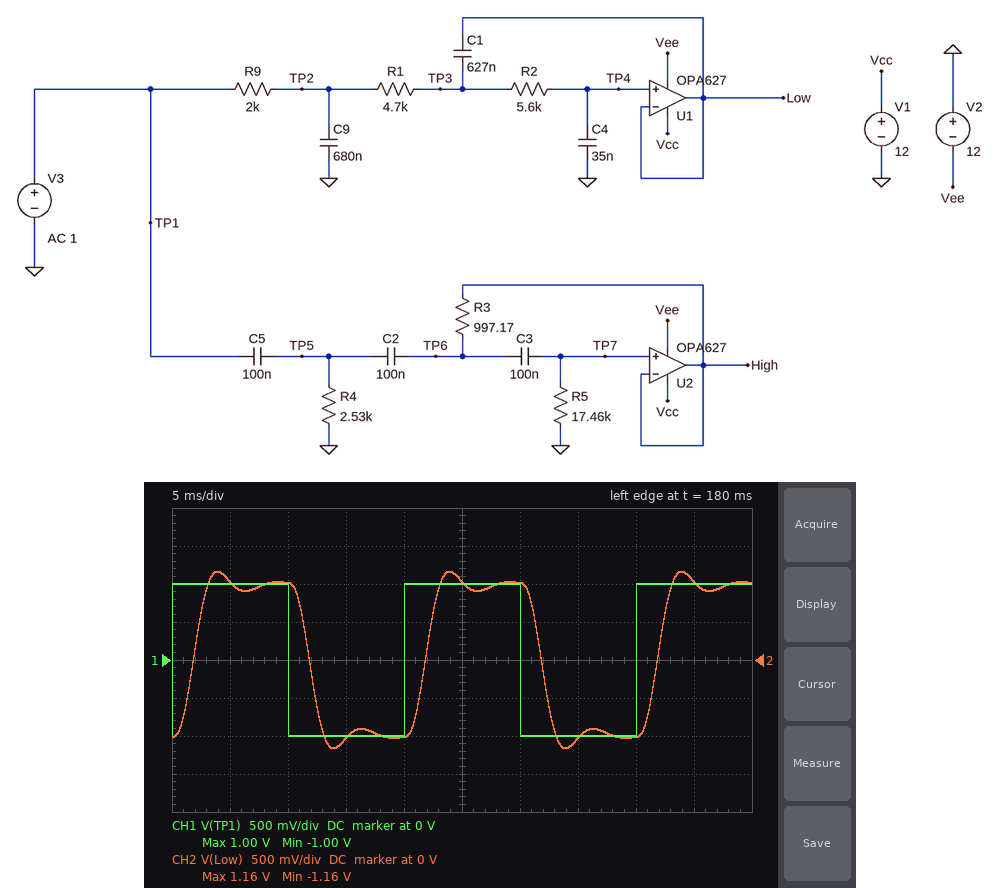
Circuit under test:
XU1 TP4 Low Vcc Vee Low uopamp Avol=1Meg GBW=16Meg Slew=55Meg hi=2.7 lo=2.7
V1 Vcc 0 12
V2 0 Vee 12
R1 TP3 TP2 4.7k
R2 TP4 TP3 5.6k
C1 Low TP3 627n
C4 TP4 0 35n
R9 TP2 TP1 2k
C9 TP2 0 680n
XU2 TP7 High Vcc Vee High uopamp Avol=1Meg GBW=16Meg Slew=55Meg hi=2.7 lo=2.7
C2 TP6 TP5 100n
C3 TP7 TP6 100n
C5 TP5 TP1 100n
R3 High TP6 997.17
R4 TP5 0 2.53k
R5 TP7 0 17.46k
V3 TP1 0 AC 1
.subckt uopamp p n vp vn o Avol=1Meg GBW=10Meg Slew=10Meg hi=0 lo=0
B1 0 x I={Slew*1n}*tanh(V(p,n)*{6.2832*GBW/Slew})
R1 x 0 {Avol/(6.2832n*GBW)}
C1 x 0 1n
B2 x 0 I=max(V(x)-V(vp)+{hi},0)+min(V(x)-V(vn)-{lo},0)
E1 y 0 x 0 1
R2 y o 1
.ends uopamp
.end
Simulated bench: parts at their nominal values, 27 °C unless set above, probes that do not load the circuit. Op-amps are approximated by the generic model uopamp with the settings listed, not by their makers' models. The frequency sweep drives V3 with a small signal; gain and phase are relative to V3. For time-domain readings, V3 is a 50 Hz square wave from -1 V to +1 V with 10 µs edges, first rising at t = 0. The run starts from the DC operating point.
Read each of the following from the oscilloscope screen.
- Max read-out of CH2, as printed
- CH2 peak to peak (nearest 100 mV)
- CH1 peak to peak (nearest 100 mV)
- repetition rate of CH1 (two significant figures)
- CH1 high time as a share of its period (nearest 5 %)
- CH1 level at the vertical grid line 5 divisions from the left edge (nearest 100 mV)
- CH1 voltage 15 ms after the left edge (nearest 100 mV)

1.16 V
2.3 V
2.0 V
50 Hz
50 %
1.0 V
-1.0 V
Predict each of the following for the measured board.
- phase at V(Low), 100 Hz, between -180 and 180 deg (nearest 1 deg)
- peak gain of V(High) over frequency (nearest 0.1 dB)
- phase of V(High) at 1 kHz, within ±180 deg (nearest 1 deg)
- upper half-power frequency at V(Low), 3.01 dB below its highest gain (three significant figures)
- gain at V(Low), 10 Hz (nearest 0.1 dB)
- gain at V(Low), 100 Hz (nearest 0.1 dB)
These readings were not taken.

-63 deg
0 dB
54 deg
211 Hz
0 dB
-0.4 dB
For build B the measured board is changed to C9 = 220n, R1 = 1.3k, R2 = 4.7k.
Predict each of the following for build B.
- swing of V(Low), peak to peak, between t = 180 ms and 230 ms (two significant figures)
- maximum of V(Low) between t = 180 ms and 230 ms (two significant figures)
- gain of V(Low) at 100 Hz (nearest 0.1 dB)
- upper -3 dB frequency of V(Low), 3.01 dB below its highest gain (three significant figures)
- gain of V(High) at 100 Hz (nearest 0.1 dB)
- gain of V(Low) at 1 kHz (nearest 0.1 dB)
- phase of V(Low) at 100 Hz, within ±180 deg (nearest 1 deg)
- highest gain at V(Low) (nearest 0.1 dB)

2.7 V
1.4 V
0.6 dB
316 Hz
-39.2 dB
-25.6 dB
-28 deg
1.4 dB
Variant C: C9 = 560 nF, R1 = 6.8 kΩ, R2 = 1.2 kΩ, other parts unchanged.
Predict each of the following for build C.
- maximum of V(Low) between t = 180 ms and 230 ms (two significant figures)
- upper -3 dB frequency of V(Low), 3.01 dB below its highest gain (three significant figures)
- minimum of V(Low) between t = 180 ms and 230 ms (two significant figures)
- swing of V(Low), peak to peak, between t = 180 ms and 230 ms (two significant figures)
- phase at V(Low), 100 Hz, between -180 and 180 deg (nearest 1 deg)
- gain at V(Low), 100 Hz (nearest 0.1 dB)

1.0 V
183 Hz
-1.0 V
2.0 V
-48 deg
-1.4 dB
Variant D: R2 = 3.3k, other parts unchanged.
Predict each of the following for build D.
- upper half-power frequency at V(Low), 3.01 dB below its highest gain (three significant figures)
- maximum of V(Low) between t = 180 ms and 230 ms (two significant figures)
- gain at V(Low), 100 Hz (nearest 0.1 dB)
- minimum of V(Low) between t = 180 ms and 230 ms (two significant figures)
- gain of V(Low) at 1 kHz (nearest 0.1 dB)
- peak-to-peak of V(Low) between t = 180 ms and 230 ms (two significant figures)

245 Hz
1.0 V
-1.3 dB
-1.0 V
-40.8 dB
2.0 V
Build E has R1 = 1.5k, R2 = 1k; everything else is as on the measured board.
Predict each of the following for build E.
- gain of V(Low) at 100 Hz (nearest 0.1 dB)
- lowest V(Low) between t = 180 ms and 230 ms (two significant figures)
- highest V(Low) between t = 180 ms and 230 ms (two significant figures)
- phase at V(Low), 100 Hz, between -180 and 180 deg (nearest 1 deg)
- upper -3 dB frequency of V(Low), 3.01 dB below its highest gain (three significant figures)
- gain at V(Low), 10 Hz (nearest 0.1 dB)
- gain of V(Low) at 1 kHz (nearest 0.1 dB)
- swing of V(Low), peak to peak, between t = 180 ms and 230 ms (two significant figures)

-2.4 dB
-1.0 V
1.0 V
-46 deg
117 Hz
0 dB
-16.8 dB
2.0 V
